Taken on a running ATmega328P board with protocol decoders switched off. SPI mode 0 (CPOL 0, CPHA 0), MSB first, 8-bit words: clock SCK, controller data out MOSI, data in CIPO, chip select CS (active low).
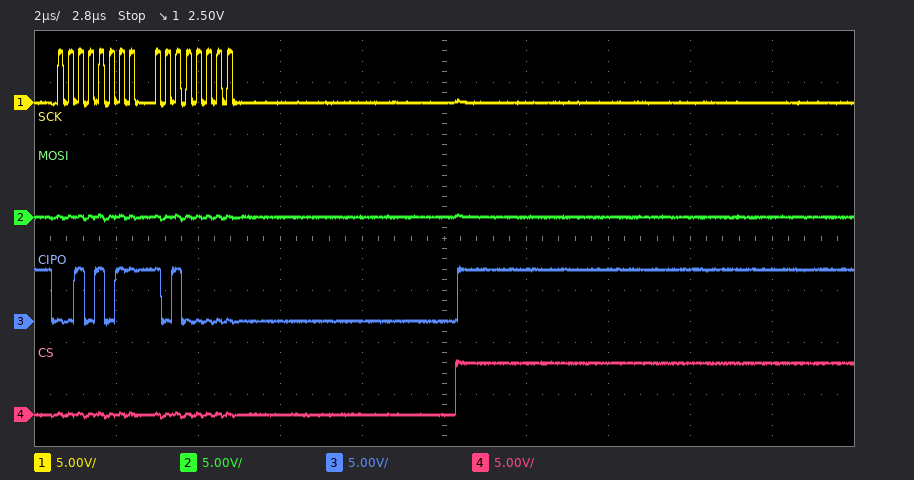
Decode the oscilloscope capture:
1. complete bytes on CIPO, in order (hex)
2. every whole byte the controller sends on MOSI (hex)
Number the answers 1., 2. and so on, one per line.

1. 2B A0
2. 00 00
